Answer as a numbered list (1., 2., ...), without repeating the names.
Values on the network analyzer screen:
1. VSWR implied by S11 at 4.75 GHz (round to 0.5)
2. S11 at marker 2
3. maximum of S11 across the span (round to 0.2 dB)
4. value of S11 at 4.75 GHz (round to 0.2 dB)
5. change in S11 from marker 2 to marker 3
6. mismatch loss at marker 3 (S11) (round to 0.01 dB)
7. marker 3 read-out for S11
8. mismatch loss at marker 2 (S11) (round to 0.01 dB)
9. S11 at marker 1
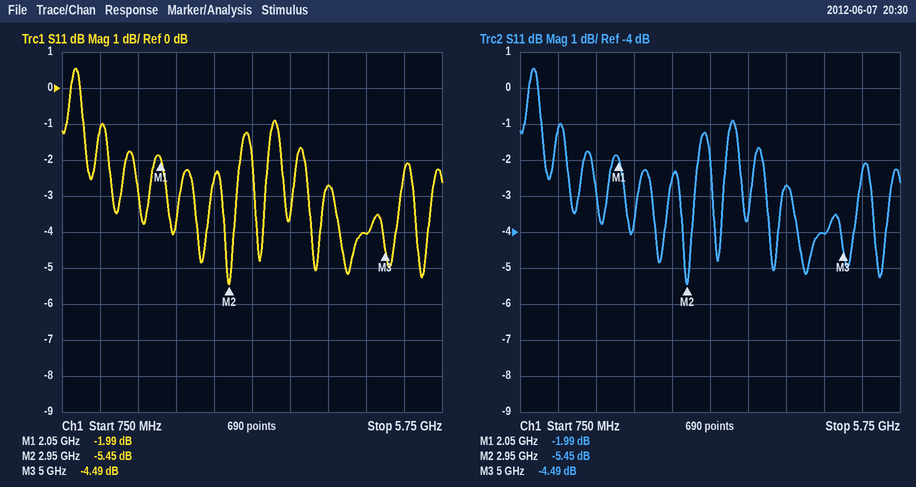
1. 4.5
2. -5.45 dB
3. 0.6 dB
4. -4.0 dB
5. 0.96 dB
6. 1.91 dB
7. -4.49 dB
8. 1.46 dB
9. -1.99 dB
